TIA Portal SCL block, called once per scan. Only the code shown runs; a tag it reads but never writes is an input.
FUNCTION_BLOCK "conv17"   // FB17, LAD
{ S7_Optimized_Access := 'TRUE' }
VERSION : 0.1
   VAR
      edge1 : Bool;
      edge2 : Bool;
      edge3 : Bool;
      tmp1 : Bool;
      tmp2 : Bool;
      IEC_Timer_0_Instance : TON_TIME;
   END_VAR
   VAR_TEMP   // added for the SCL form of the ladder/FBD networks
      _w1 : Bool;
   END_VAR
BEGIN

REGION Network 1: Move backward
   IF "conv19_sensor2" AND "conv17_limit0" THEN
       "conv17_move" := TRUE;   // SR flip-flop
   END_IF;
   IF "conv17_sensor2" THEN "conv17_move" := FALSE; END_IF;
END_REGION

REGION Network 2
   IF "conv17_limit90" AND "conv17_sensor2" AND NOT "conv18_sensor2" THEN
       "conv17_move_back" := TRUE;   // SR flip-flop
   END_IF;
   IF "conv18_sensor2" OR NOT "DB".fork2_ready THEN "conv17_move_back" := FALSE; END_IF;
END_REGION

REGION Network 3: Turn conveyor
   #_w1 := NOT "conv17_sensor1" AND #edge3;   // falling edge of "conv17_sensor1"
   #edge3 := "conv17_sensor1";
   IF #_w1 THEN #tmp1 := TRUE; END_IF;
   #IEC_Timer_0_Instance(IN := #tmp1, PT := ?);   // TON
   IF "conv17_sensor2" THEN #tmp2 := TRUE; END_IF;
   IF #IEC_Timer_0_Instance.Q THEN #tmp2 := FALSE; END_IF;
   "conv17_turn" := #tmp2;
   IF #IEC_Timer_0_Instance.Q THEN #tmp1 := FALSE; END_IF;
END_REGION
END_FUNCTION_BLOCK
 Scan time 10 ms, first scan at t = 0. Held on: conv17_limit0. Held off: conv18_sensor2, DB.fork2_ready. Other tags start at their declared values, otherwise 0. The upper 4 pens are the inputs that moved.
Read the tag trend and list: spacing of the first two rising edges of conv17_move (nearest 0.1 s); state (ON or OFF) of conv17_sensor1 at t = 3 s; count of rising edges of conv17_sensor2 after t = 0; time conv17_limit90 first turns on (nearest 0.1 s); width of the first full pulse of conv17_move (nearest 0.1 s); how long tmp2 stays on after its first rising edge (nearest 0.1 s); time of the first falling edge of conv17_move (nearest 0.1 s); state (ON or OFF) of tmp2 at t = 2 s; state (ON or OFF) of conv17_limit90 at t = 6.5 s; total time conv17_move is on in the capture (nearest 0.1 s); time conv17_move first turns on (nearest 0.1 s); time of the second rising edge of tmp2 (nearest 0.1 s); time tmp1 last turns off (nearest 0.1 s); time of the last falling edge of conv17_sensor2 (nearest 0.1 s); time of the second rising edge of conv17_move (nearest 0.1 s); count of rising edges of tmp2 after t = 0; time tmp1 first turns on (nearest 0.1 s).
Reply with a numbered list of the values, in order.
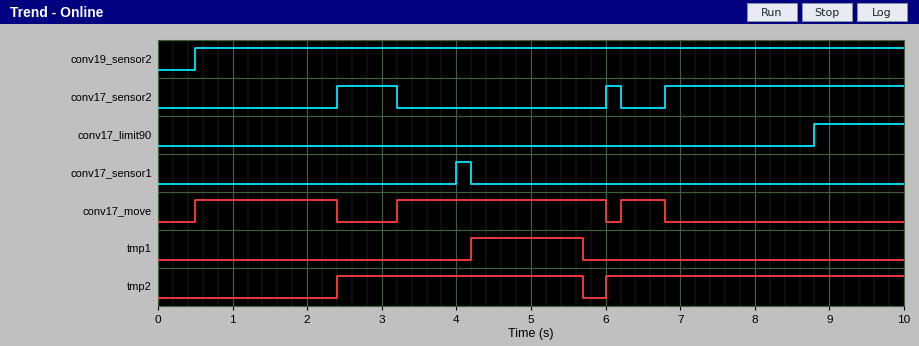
1. 2.7 s
2. OFF
3. 3
4. 8.8 s
5. 1.9 s
6. 3.3 s
7. 2.4 s
8. OFF
9. OFF
10. 5.3 s
11. 0.5 s
12. 6.0 s
13. 5.7 s
14. 6.2 s
15. 3.2 s
16. 2
17. 4.2 s
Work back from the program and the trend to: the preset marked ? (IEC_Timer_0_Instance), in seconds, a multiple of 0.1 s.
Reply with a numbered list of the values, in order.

1. 1.5 s
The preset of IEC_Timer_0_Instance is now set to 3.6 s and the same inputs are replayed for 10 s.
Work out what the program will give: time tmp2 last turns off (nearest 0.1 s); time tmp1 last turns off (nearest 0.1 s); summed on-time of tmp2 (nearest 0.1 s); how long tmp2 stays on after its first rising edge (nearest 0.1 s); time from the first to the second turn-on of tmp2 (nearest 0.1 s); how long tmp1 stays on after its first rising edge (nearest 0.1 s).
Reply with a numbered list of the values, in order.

1. 7.8 s
2. 7.8 s
3. 7.6 s
4. 5.4 s
5. 5.4 s
6. 3.6 s
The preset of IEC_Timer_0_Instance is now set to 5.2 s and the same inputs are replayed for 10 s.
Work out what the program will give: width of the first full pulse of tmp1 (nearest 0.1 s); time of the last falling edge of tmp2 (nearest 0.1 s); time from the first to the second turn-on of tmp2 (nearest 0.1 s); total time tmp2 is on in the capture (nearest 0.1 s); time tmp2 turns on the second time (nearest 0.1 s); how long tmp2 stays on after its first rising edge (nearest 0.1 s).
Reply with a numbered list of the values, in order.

1. 5.2 s
2. 9.4 s
3. 7.0 s
4. 7.6 s
5. 9.4 s
6. 7.0 s
